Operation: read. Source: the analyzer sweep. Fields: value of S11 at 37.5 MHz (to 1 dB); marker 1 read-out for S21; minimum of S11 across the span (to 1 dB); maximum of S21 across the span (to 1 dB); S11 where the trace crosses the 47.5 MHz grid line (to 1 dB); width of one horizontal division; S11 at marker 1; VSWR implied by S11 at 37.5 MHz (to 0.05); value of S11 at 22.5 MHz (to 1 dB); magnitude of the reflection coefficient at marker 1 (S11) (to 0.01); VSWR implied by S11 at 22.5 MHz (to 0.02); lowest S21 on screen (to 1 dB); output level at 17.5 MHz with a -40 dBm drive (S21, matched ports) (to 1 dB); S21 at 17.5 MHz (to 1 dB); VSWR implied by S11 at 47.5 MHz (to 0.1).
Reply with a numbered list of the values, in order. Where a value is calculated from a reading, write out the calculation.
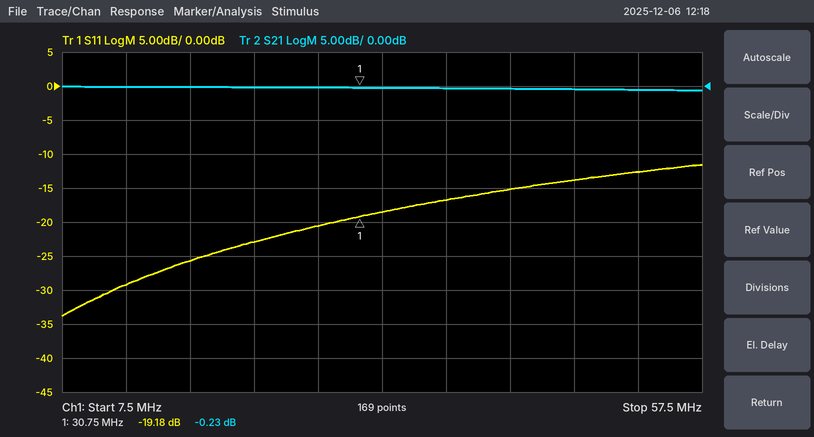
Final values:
1. -17 dB
2. -0.23 dB
3. -34 dB
4. 0 dB
5. -14 dB
6. 5 MHz
7. -19.18 dB
8. |Γ| = 10^(-17/20) = 0.1413; VSWR = (1 + 0.1413)/(1 − 0.1413) ≈ 1.33, so 1.35 to the nearest 0.05
9. -23 dB
10. 10^(-19.18/20) ≈ 0.11
11. |Γ| = 10^(-23/20) = 0.0708; VSWR = (1 + 0.0708)/(1 − 0.0708) ≈ 1.15, so 1.16 to the nearest 0.02
12. -1 dB
13. -40 dBm + (0 dB) = -40 dBm
14. 0 dB
15. |Γ| = 10^(-14/20) = 0.1995; VSWR = (1 + 0.1995)/(1 − 0.1995) ≈ 1.5
